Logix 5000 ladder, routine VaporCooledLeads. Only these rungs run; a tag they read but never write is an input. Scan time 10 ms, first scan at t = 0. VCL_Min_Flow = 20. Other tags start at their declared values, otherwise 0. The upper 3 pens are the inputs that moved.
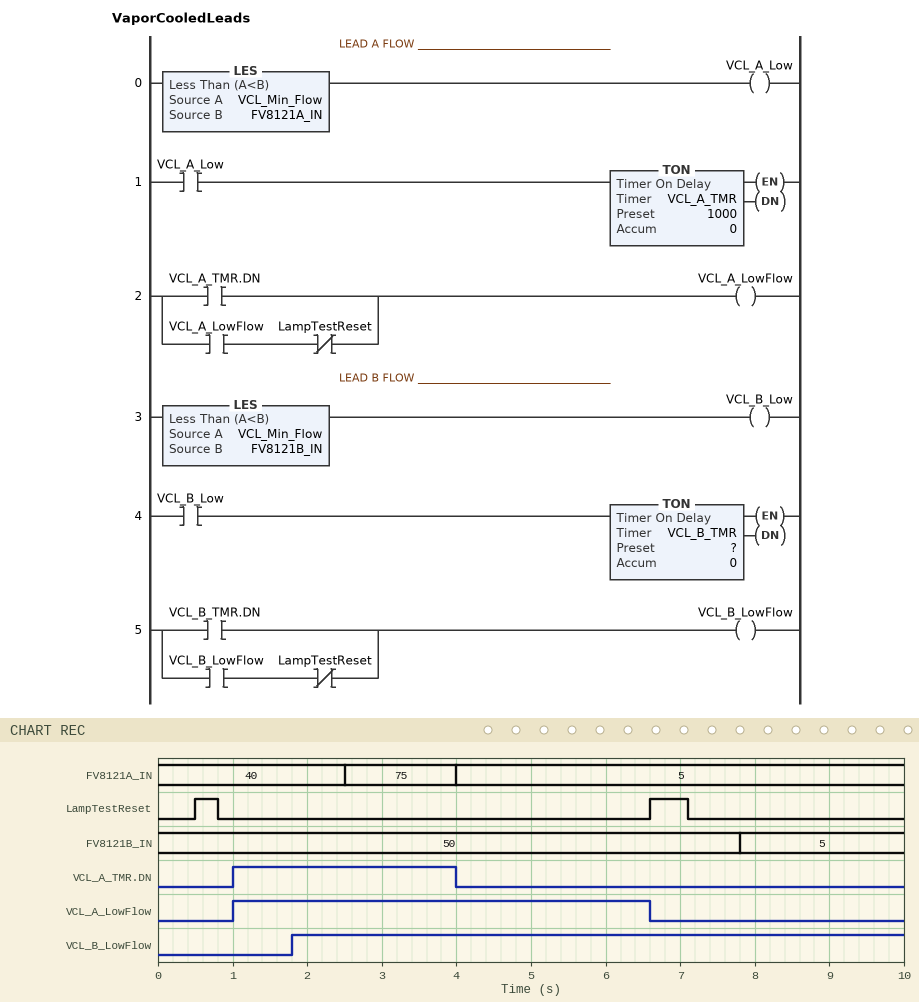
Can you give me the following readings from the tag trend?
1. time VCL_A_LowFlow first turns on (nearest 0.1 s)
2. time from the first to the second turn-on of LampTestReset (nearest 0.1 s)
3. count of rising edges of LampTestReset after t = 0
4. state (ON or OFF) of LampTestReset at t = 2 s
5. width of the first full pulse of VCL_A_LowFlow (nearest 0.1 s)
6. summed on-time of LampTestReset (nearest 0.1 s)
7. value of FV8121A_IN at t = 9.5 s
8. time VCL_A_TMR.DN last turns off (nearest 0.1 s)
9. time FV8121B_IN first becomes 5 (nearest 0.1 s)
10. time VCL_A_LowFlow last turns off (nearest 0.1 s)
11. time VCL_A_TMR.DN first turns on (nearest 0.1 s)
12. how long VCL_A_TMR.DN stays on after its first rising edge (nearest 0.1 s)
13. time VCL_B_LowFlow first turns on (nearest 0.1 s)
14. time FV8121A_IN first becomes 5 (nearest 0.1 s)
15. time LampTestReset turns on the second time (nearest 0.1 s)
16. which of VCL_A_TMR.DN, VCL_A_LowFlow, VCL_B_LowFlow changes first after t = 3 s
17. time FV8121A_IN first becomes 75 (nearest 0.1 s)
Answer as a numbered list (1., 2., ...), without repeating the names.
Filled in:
1. 1.0 s
2. 6.1 s
3. 2
4. OFF
5. 5.6 s
6. 0.8 s
7. 5
8. 4.0 s
9. 7.8 s
10. 6.6 s
11. 1.0 s
12. 3.0 s
13. 1.8 s
14. 4.0 s
15. 6.6 s
16. VCL_A_TMR.DN
17. 2.5 s
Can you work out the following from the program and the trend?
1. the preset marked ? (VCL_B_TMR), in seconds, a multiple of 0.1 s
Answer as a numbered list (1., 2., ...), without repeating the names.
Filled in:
1. 1.8 s
